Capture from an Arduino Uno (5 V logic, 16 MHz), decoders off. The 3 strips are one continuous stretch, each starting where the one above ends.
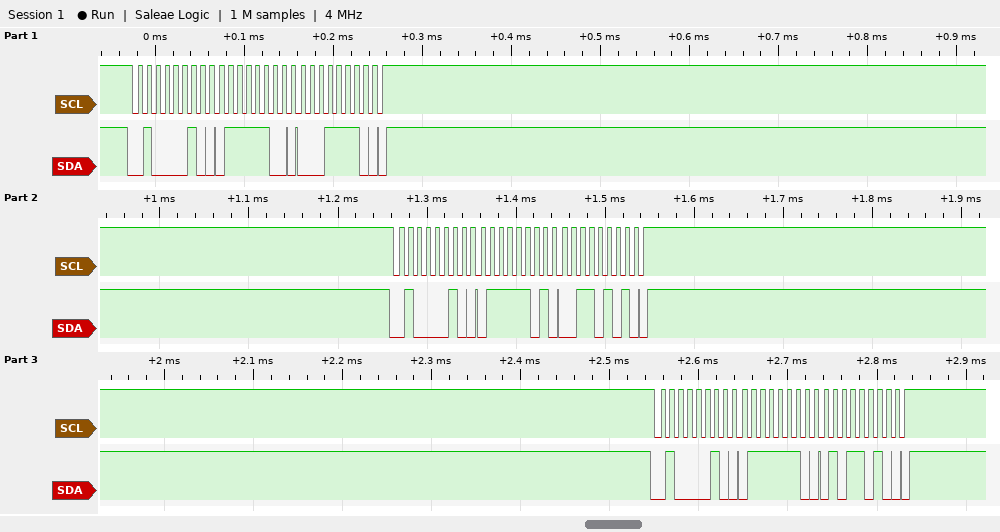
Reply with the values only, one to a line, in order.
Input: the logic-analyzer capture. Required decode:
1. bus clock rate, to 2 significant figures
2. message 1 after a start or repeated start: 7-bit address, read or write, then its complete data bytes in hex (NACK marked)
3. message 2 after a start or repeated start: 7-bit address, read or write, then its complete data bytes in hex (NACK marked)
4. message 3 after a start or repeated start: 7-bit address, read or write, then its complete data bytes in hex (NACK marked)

100 kHz
0x21 write: 7C 1E
0x21 write: 7D 35
0x21 write: 7E 5A
